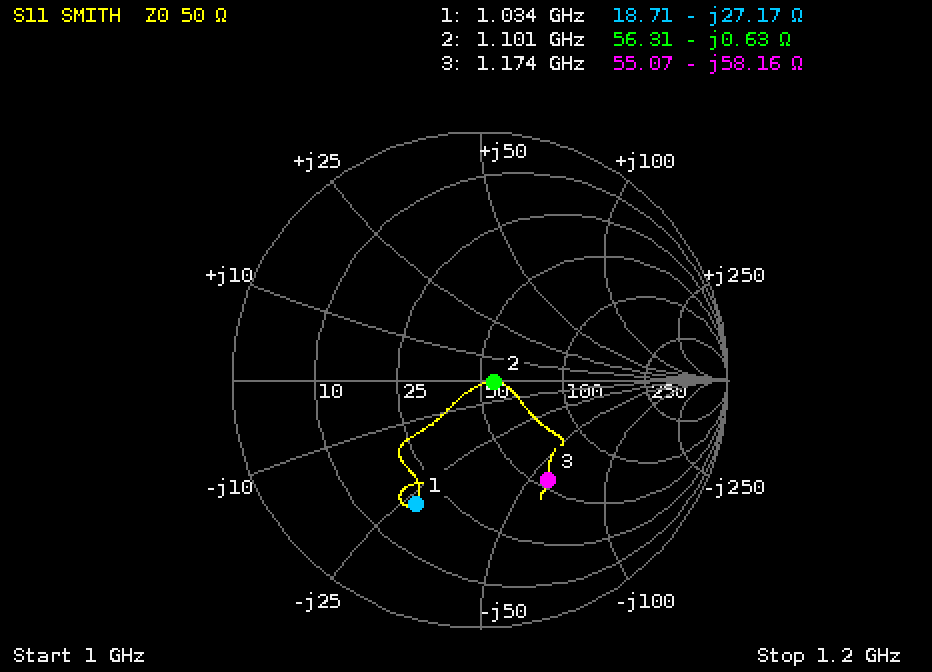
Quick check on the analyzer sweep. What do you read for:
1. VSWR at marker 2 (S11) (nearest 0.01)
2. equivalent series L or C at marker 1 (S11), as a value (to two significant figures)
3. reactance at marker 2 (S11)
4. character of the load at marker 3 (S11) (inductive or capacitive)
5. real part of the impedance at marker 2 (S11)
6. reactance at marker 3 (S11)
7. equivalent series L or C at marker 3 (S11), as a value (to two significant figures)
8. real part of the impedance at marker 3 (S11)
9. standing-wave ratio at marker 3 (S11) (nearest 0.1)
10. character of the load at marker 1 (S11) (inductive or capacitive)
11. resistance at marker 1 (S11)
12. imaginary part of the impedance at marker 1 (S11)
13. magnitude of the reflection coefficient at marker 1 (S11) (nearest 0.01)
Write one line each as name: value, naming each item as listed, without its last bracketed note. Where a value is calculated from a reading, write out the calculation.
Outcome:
VSWR at marker 2 (S11): 1.13
equivalent series L or C at marker 1 (S11), as a value: C = 1/(2π × 1.034 GHz × 27.17 Ω) ≈ 5.7 pF
reactance at marker 2: -0.63 Ω
character of the load at marker 3 (S11): capacitive
real part of the impedance at marker 2: 56.31 Ω
reactance at marker 3: -58.16 Ω
equivalent series L or C at marker 3 (S11), as a value: C = 1/(2π × 1.174 GHz × 58.16 Ω) ≈ 2.3 pF
real part of the impedance at marker 3: 55.07 Ω
standing-wave ratio at marker 3 (S11): 2.9
character of the load at marker 1 (S11): capacitive
resistance at marker 1: 18.71 Ω
imaginary part of the impedance at marker 1: -27.17 Ω
magnitude of the reflection coefficient at marker 1 (S11): 0.56
